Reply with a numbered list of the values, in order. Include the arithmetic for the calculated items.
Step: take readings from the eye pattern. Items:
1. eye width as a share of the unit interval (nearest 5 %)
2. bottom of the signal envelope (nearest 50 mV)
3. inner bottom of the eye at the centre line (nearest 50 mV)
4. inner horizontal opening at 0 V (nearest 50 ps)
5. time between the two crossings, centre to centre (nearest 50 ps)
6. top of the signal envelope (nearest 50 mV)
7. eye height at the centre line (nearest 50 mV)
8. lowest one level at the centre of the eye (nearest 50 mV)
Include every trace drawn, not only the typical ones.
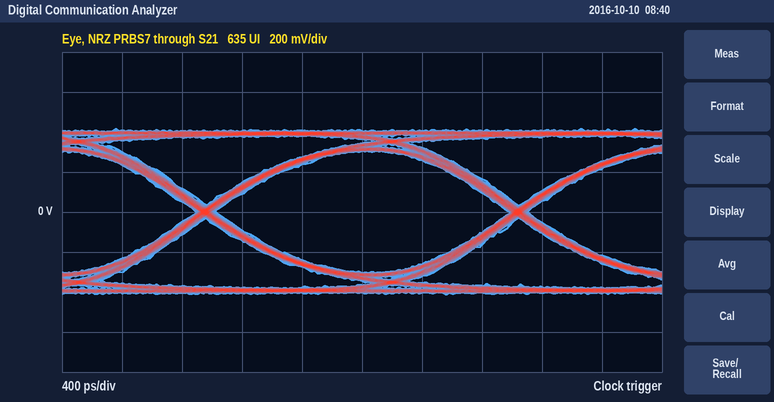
1. 1.95 ns / 2.10 ns ≈ 92.9 %, so 95 % to the nearest 5 %
2. -400 mV
3. -300 mV
4. 1.95 ns
5. 2.10 ns
6. 400 mV
7. 600 mV
8. 300 mV
